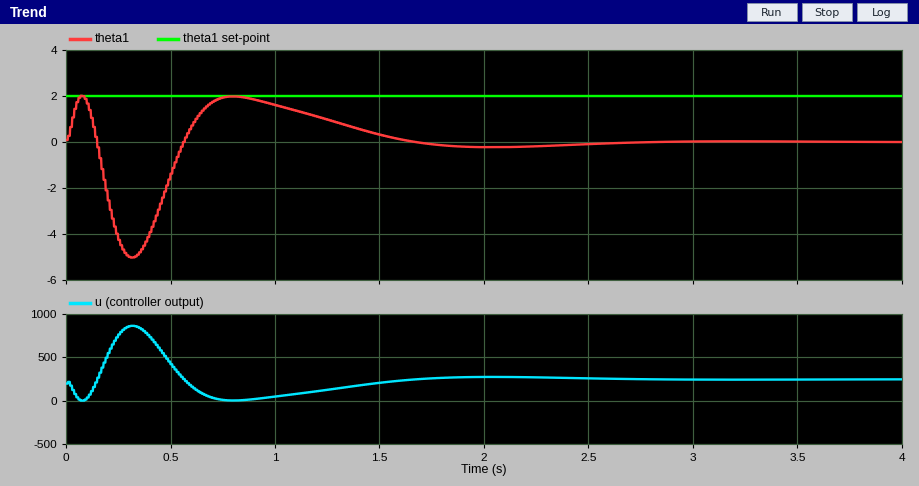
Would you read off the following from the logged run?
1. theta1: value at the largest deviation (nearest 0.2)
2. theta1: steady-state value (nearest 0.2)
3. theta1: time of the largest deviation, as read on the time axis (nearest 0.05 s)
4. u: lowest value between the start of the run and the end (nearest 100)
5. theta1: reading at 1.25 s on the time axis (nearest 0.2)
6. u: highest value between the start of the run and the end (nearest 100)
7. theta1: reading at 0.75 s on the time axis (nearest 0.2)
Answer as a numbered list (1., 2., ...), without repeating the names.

1. -5.0
2. 0.0
3. 0.30 s
4. 0
5. 1.0
6. 900
7. 2.0
